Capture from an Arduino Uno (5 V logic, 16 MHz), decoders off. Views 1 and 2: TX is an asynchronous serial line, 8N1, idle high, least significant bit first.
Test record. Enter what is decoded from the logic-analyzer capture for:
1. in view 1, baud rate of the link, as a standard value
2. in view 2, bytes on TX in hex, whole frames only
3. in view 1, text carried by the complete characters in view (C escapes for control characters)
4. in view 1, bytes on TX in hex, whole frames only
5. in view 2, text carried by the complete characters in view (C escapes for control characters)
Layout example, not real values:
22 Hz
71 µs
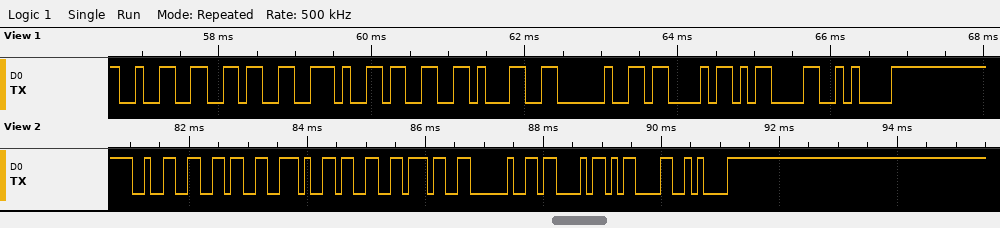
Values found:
9600 baud
32 36 2E 33 37 20 43 0D 0A
"26.31 C\r\n"
32 36 2E 33 31 20 43 0D 0A
"26.37 C\r\n"
